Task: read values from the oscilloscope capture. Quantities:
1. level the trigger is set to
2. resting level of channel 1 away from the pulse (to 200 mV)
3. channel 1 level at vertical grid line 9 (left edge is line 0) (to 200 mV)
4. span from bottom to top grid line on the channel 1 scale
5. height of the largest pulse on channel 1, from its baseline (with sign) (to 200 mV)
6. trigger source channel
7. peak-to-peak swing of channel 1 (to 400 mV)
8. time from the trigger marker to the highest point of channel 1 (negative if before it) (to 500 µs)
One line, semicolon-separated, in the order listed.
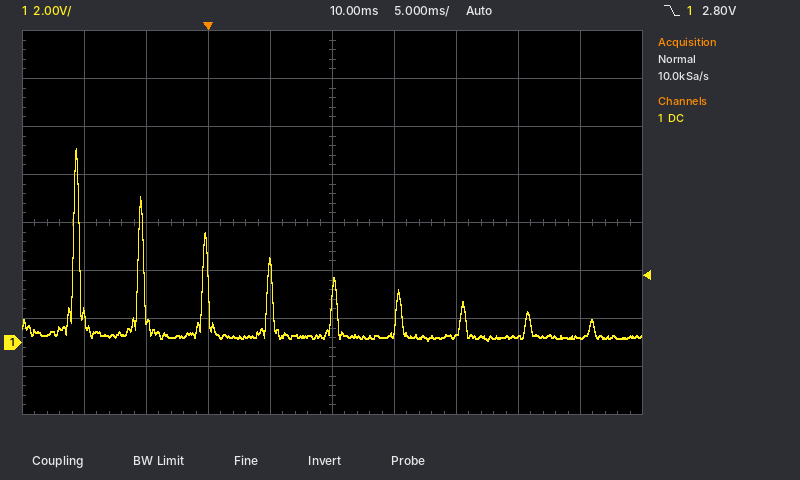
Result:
2.80 V; 200 mV; 200 mV; 16 V; +7.8 V; channel 1; 8.0 V; -10.5 ms
